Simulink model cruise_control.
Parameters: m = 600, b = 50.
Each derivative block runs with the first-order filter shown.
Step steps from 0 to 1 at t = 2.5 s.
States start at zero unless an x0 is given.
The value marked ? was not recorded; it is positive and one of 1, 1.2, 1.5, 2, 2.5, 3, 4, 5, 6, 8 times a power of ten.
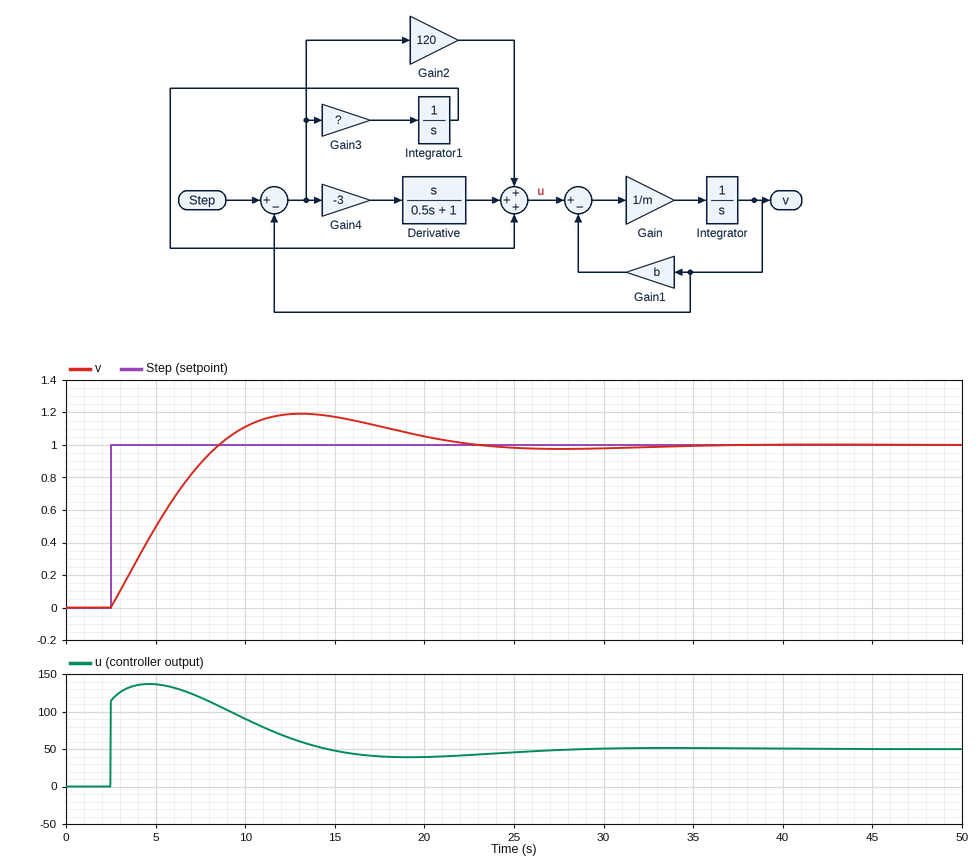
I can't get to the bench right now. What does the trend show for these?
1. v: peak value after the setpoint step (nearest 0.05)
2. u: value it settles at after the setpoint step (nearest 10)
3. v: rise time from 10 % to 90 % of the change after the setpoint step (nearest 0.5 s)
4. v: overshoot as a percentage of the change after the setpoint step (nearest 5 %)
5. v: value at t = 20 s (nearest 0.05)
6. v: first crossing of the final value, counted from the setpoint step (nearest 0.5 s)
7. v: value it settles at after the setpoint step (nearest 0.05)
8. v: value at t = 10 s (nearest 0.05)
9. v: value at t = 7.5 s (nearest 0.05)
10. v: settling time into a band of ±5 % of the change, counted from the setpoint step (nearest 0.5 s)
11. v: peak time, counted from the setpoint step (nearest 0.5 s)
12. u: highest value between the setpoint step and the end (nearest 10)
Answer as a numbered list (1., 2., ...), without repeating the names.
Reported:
1. 1.20
2. 50
3. 4.5 s
4. 20 %
5. 1.05
6. 6.0 s
7. 1.00
8. 1.10
9. 0.90
10. 17.5 s
11. 10.5 s
12. 140
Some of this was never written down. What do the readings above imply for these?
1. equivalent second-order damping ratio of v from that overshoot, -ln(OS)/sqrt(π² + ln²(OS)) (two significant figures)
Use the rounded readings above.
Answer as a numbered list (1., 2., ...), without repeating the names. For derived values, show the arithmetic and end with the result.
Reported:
1. ln(0.2) = -1.609; 1.609 / sqrt(9.870 + 2.590) = 0.46
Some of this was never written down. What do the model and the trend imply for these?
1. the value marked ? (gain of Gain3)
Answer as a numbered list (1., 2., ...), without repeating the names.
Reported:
1. 40
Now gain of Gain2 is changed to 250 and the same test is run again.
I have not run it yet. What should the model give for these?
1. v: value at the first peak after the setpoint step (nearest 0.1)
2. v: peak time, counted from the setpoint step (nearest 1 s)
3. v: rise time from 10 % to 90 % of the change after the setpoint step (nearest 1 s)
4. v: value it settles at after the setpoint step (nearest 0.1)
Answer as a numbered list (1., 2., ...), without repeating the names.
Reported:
1. 1.1
2. 10 s
3. 4 s
4. 1.0
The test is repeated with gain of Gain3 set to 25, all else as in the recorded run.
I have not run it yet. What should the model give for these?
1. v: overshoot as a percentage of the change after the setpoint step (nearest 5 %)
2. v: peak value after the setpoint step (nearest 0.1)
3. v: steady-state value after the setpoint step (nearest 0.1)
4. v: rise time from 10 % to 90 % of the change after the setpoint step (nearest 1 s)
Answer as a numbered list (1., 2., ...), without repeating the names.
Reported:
1. 10 %
2. 1.1
3. 1.0
4. 6 s
